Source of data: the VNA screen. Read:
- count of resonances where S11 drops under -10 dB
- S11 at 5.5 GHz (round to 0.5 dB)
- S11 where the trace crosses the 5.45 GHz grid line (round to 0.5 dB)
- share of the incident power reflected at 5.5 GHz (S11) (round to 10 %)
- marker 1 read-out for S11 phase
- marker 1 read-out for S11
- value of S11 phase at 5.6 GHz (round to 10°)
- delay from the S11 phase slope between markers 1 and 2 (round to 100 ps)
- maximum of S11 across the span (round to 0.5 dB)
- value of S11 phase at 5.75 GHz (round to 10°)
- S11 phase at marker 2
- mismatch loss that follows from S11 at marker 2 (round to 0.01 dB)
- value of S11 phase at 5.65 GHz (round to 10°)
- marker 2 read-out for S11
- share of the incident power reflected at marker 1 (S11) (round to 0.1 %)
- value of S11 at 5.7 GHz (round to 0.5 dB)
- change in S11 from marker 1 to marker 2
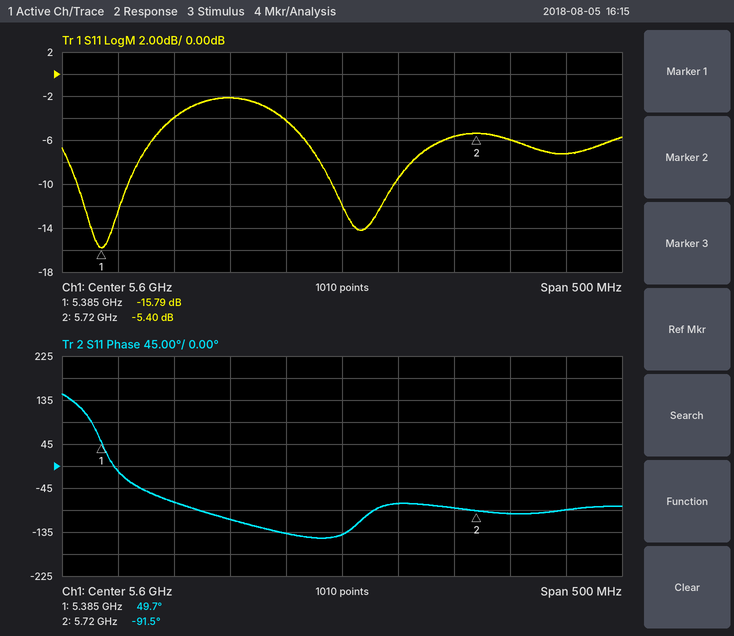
2
-2.0 dB
-4.0 dB
60 %
49.7°
-15.79 dB
-140°
1.2 ns
-2.0 dB
-100°
-91.5°
1.48 dB
-80°
-5.40 dB
2.6 %
-5.5 dB
10.39 dB
